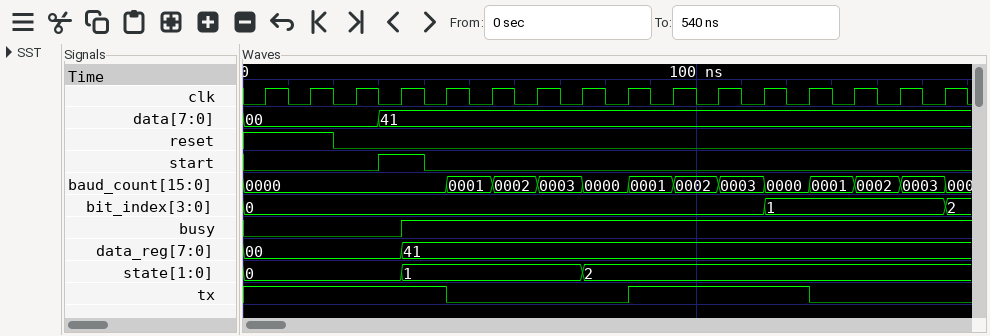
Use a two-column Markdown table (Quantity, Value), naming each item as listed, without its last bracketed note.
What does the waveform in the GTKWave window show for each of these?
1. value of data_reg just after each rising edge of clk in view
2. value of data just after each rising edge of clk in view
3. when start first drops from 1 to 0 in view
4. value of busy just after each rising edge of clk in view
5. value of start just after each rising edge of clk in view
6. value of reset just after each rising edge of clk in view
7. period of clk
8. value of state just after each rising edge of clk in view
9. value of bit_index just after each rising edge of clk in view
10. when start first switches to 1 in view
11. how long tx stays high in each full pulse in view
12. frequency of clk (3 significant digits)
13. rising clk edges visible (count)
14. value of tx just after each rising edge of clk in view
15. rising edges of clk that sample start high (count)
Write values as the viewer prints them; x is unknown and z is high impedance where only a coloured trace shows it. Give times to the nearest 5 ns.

| Quantity | Value |
|---|---|
| value of data_reg just after each rising edge of clk in view | 00, 00, 00, 41, 41, 41, 41, 41, 41, 41, 41, 41, 41, 41, 41, 41 |
| value of data just after each rising edge of clk in view | 00, 00, 00, 41, 41, 41, 41, 41, 41, 41, 41, 41, 41, 41, 41, 41 |
| when start first drops from 1 to 0 in view | 40 ns |
| value of busy just after each rising edge of clk in view | 0 0 0 1 1 1 1 1 1 1 1 1 1 1 1 1 |
| value of start just after each rising edge of clk in view | 0 0 0 1 0 0 0 0 0 0 0 0 0 0 0 0 |
| value of reset just after each rising edge of clk in view | 1 1 0 0 0 0 0 0 0 0 0 0 0 0 0 0 |
| period of clk | 10 ns |
| value of state just after each rising edge of clk in view | 0, 0, 0, 1, 1, 1, 1, 2, 2, 2, 2, 2, 2, 2, 2, 2 |
| value of bit_index just after each rising edge of clk in view | 0, 0, 0, 0, 0, 0, 0, 0, 0, 0, 0, 1, 1, 1, 1, 2 |
| when start first switches to 1 in view | 30 ns |
| how long tx stays high in each full pulse in view | 40 ns |
| frequency of clk | 100 MHz |
| rising clk edges visible | 16 |
| value of tx just after each rising edge of clk in view | 1 1 1 1 0 0 0 0 1 1 1 1 0 0 0 0 |
| rising edges of clk that sample start high | 1 |
